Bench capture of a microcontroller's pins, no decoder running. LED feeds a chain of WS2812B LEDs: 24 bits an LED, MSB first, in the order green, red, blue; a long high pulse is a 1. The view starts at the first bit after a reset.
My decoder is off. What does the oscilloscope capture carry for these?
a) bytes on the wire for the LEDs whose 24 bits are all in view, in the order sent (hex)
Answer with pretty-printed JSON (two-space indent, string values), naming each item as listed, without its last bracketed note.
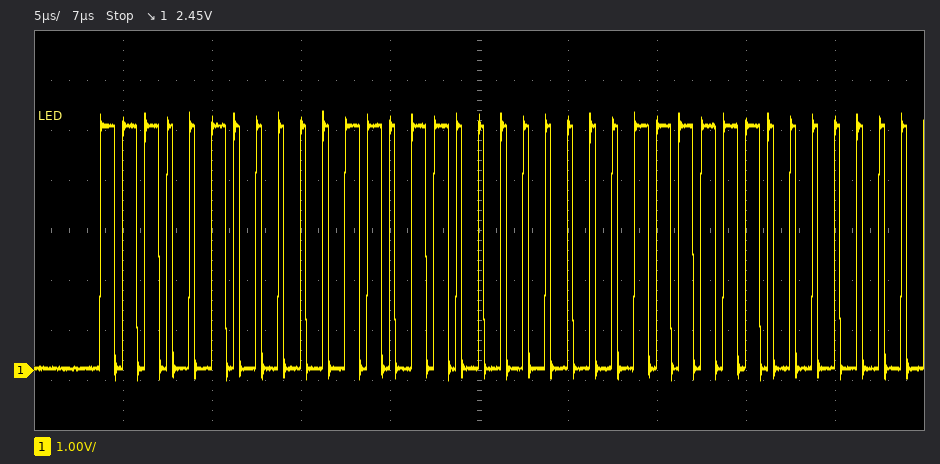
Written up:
{
  "bytes on the wire for the LEDs whose 24 bits are all in view, in the order sent": "E4 1B 00"
}
